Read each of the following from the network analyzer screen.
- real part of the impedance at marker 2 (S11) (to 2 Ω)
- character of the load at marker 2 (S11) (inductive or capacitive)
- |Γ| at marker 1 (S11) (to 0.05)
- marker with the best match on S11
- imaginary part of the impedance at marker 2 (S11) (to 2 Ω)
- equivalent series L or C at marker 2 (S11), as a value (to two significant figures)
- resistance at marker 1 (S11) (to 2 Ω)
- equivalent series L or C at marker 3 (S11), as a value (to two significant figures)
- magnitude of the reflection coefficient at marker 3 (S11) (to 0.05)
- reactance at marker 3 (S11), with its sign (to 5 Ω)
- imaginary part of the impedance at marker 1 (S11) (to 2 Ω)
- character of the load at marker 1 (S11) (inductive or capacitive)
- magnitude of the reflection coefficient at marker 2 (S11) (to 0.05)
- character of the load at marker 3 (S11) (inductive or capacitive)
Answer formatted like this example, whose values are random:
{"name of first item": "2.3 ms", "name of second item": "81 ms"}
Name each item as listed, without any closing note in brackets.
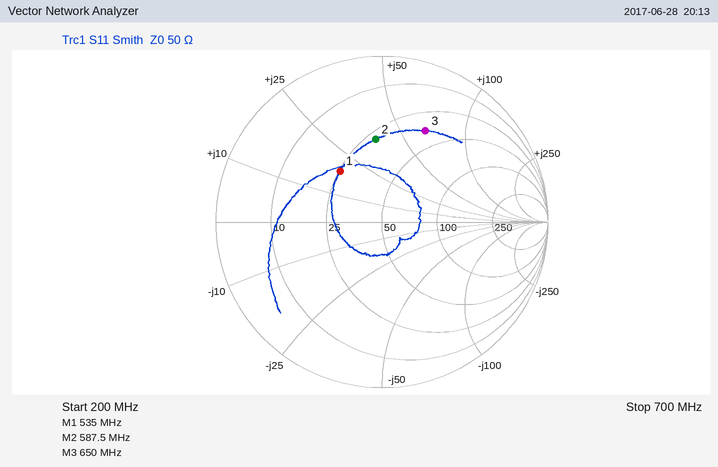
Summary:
{"real part of the impedance at marker 2 (S11)": "28 Ω", "character of the load at marker 2 (S11)": "inductive", "|Γ| at marker 1 (S11)": "0.40", "marker with the best match on S11": "marker 1", "imaginary part of the impedance at marker 2 (S11)": "+38 Ω", "equivalent series L or C at marker 2 (S11), as a value": "10 nH", "resistance at marker 1 (S11)": "26 Ω", "equivalent series L or C at marker 3 (S11), as a value": "16 nH", "magnitude of the reflection coefficient at marker 3 (S11)": "0.60", "reactance at marker 3 (S11), with its sign": "+65 Ω", "imaginary part of the impedance at marker 1 (S11)": "+18 Ω", "character of the load at marker 1 (S11)": "inductive", "magnitude of the reflection coefficient at marker 2 (S11)": "0.50", "character of the load at marker 3 (S11)": "inductive"}
